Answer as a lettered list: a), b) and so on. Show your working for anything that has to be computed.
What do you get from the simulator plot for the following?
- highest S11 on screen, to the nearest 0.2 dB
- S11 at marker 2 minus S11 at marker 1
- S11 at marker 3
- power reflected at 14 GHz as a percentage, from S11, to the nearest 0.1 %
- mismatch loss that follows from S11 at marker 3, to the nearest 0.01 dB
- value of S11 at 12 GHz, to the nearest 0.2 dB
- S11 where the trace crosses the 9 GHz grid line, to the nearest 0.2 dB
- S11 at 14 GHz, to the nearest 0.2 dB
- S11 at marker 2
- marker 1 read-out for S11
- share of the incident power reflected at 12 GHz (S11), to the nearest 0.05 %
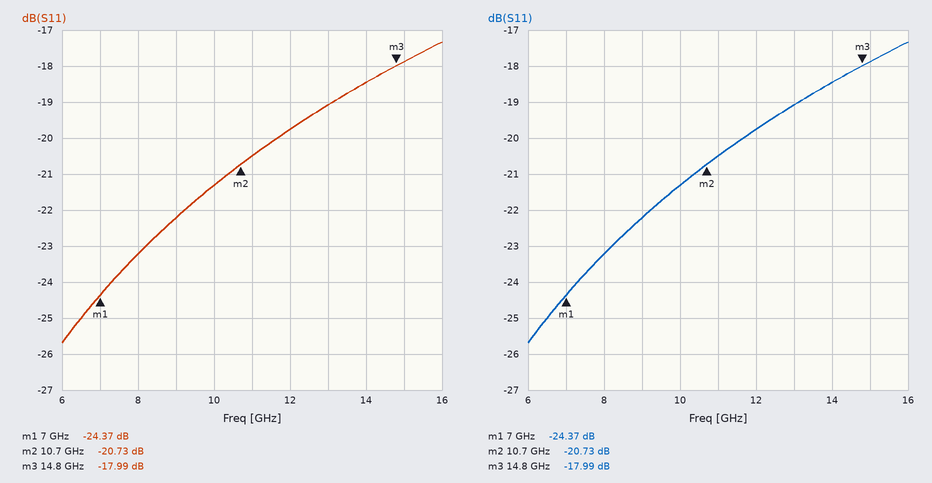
a) -17.4 dB
b) -20.73 − (-24.37) = 3.64 dB
c) -17.99 dB
d) 10^(-18.4/10) ≈ 1.4 %
e) −10 log10(1 − 10^(-17.99/10)) ≈ 0.07 dB
f) -19.8 dB
g) -22.2 dB
h) -18.4 dB
i) -20.73 dB
j) -24.37 dB
k) 10^(-19.8/10) ≈ 1.05 %
